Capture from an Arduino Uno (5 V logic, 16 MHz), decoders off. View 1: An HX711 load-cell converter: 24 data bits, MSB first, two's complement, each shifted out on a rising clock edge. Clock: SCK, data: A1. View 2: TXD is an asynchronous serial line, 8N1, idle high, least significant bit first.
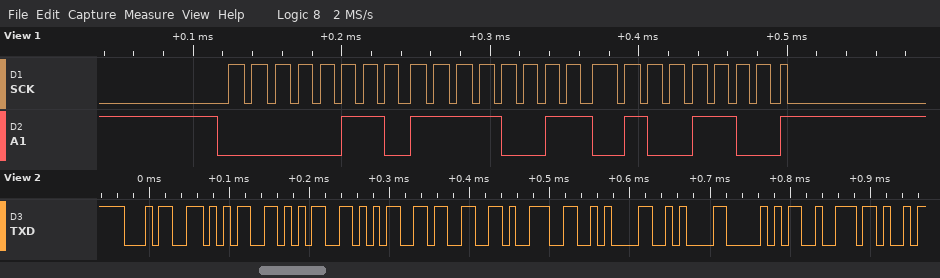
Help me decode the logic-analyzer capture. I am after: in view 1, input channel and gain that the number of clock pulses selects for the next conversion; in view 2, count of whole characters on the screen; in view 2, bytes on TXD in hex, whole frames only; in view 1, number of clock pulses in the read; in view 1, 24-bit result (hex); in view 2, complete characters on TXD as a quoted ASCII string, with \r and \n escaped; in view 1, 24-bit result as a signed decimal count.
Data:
channel A, gain 128
10
34 35 35 35 33 39 0A 0A 50 72
25
0x06F34C
"455539\n\nPr"
455500
